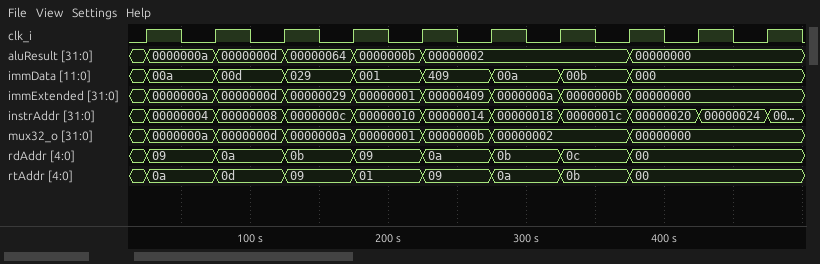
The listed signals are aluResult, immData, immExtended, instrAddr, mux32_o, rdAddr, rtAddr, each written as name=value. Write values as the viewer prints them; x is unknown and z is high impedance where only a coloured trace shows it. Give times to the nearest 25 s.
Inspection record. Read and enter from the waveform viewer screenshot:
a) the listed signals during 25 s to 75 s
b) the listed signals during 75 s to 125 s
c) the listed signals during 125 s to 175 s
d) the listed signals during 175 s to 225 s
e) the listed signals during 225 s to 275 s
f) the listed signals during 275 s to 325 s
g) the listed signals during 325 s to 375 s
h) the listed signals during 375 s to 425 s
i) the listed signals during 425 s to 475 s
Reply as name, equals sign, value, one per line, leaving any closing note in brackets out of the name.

the listed signals during 25 s to 75 s = aluResult=0000000a, immData=00a, immExtended=0000000a, instrAddr=00000004, mux32_o=0000000a, rdAddr=09, rtAddr=0a
the listed signals during 75 s to 125 s = aluResult=0000000d, immData=00d, immExtended=0000000d, instrAddr=00000008, mux32_o=0000000d, rdAddr=0a, rtAddr=0d
the listed signals during 125 s to 175 s = aluResult=00000064, immData=029, immExtended=00000029, instrAddr=0000000c, mux32_o=0000000a, rdAddr=0b, rtAddr=09
the listed signals during 175 s to 225 s = aluResult=0000000b, immData=001, immExtended=00000001, instrAddr=00000010, mux32_o=00000001, rdAddr=09, rtAddr=01
the listed signals during 225 s to 275 s = aluResult=00000002, immData=409, immExtended=00000409, instrAddr=00000014, mux32_o=0000000b, rdAddr=0a, rtAddr=09
the listed signals during 275 s to 325 s = aluResult=00000002, immData=00a, immExtended=0000000a, instrAddr=00000018, mux32_o=00000002, rdAddr=0b, rtAddr=0a
the listed signals during 325 s to 375 s = aluResult=00000002, immData=00b, immExtended=0000000b, instrAddr=0000001c, mux32_o=00000002, rdAddr=0c, rtAddr=0b
the listed signals during 375 s to 425 s = aluResult=00000000, immData=000, immExtended=00000000, instrAddr=00000020, mux32_o=00000000, rdAddr=00, rtAddr=00
the listed signals during 425 s to 475 s = aluResult=00000000, immData=000, immExtended=00000000, instrAddr=00000024, mux32_o=00000000, rdAddr=00, rtAddr=00
